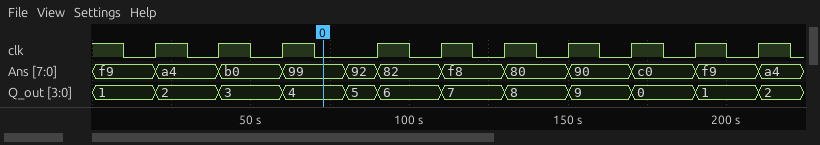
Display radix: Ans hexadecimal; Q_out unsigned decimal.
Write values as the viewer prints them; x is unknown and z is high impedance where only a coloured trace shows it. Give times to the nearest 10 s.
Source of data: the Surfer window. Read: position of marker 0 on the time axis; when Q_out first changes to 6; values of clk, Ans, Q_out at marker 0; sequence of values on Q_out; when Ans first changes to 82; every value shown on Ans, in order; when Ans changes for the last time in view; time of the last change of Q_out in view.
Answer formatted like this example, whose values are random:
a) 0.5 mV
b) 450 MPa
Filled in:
a) 70 s
b) 90 s
c) clk=0, Ans=99, Q_out=4
d) 1, 2, 3, 4, 5, 6, 7, 8, 9, 0, 1, 2
e) 90 s
f) f9, a4, b0, 99, 92, 82, f8, 80, 90, c0, f9, a4
g) 210 s
h) 210 s
